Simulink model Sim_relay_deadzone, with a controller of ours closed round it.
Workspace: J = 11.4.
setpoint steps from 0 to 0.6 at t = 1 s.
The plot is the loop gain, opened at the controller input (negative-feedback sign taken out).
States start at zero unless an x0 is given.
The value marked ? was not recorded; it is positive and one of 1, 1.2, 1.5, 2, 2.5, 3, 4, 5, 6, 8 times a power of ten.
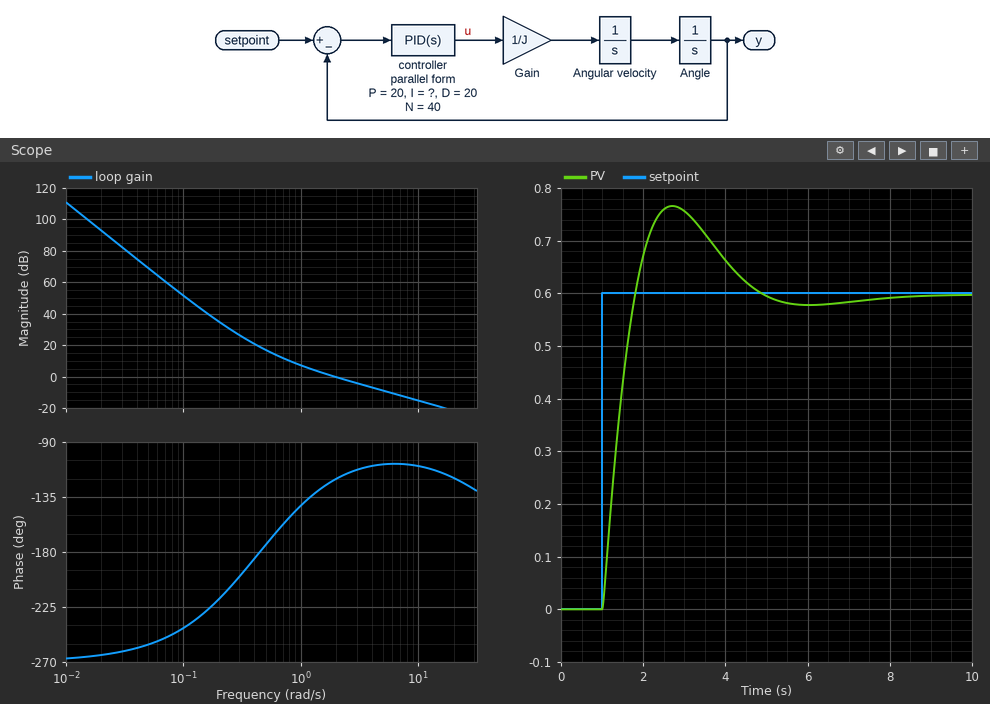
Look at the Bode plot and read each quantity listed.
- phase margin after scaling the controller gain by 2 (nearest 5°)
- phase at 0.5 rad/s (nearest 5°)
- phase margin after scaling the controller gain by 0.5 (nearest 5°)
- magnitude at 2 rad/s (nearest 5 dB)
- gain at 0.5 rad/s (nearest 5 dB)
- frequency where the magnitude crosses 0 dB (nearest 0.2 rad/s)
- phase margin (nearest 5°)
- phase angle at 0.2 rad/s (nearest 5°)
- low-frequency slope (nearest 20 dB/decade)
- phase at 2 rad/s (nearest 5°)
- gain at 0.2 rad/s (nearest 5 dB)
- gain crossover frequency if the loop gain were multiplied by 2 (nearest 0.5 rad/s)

70°
-175°
40°
0 dB
15 dB
2.0 rad/s
60°
-220°
-60 dB/decade
-120°
35 dB
3.5 rad/s
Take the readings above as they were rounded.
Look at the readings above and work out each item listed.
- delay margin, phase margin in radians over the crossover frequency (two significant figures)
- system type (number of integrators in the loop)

0.52 s
3
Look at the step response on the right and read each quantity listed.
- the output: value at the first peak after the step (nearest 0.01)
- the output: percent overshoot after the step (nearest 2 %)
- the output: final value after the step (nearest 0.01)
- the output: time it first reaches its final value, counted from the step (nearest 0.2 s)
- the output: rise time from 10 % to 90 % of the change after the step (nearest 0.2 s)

0.77
28 %
0.60
0.8 s
0.6 s
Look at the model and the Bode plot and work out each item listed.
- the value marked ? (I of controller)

4
